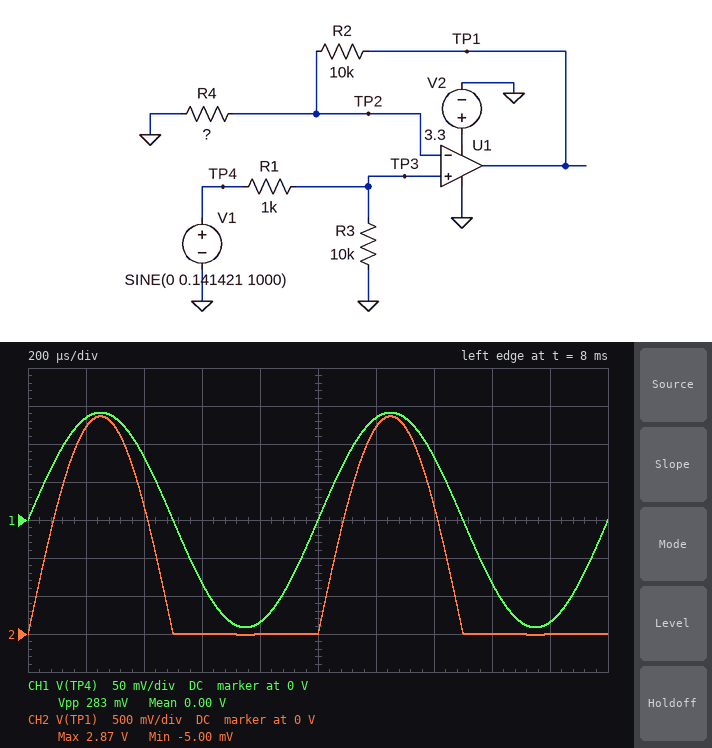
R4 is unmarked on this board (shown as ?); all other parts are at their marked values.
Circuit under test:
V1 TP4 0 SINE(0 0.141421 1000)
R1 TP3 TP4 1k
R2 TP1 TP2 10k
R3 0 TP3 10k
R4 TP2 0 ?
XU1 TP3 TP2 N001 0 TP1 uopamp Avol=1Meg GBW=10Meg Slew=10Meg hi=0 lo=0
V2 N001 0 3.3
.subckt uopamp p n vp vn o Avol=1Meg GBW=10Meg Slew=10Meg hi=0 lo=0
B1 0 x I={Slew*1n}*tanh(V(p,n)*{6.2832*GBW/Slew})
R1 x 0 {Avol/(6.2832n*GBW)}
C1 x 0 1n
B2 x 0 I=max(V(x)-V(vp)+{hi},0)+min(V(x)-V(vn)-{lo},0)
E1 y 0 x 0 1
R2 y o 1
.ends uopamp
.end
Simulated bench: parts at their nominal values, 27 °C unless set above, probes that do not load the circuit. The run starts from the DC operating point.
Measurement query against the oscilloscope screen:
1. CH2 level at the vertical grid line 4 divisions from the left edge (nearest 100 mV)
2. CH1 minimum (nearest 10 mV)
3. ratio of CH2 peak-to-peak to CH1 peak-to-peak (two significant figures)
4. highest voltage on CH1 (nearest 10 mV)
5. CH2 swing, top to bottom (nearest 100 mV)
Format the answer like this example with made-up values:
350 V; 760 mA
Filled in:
0 V; -140 mV; 10; 140 mV; 2.9 V
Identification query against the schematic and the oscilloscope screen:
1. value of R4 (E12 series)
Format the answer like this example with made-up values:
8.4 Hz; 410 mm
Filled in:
470 Ω
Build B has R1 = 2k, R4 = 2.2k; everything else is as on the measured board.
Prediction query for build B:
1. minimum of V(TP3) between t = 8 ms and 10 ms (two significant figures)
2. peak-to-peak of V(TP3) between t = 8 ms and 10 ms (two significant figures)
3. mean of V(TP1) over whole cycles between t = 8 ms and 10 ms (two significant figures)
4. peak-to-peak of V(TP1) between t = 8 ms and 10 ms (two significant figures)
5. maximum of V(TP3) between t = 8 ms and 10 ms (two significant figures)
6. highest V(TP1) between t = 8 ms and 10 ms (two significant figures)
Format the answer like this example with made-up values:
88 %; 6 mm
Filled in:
-120 mV; 240 mV; 210 mV; 660 mV; 120 mV; 650 mV
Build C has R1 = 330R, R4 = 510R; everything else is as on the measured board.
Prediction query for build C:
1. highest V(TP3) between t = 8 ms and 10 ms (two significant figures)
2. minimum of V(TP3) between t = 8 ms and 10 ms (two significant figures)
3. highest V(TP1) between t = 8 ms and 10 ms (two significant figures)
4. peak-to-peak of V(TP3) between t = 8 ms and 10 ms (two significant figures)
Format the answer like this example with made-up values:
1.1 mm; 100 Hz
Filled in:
140 mV; -140 mV; 2.8 V; 270 mV
